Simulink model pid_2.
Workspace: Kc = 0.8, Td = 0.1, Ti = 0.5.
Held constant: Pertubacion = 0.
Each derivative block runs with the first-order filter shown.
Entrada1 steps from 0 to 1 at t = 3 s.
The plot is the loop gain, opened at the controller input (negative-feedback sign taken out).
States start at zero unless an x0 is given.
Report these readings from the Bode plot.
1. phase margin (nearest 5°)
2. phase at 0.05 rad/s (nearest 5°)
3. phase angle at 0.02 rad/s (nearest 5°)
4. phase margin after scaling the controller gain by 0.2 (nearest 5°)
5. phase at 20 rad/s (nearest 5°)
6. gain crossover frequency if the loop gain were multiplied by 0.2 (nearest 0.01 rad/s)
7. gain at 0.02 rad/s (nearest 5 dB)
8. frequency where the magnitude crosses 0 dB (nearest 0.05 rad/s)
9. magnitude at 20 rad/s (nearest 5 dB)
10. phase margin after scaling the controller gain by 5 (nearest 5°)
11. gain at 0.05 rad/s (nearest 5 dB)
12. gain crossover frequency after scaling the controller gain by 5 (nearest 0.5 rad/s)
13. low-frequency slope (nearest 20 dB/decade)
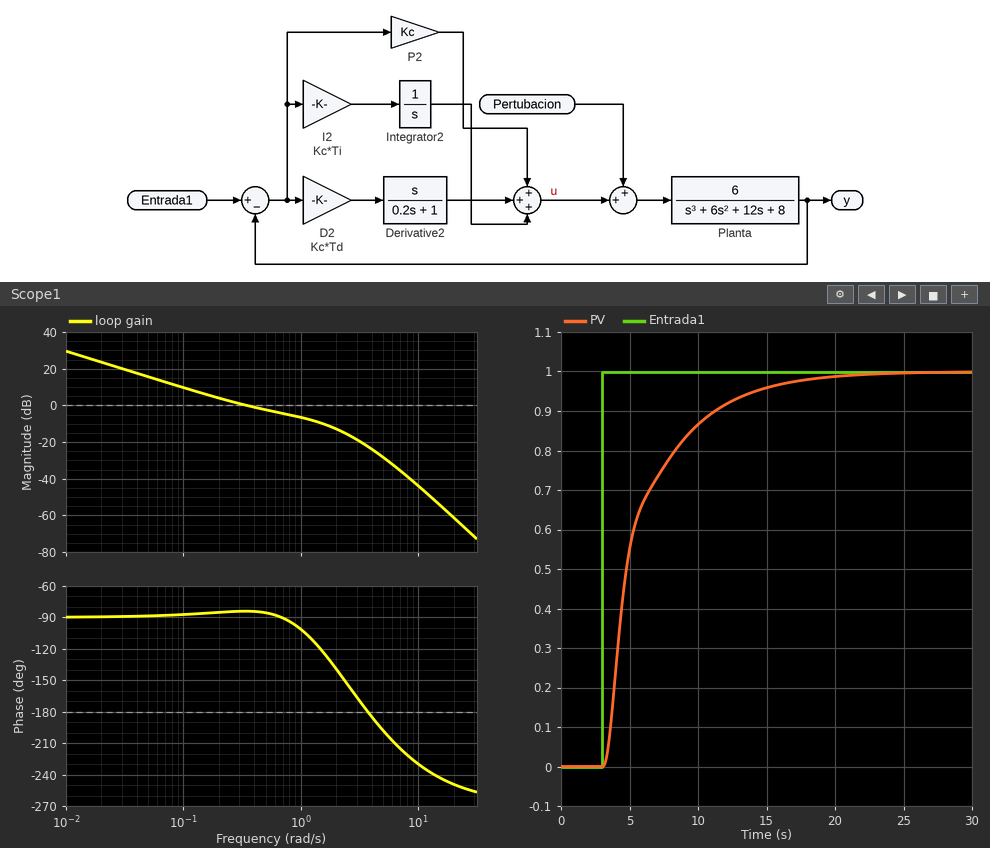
95°
-90°
-90°
90°
-250°
0.06 rad/s
25 dB
0.35 rad/s
-60 dB
35°
15 dB
2.0 rad/s
-20 dB/decade
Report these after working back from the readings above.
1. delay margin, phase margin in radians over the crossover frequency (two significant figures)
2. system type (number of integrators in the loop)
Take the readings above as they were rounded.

4.7 s
1
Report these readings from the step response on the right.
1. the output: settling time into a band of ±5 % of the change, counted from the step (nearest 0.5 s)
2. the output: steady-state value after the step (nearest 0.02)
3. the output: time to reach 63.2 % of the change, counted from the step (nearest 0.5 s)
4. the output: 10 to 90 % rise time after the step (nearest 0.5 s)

11.0 s
1.00
2.5 s
7.5 s
